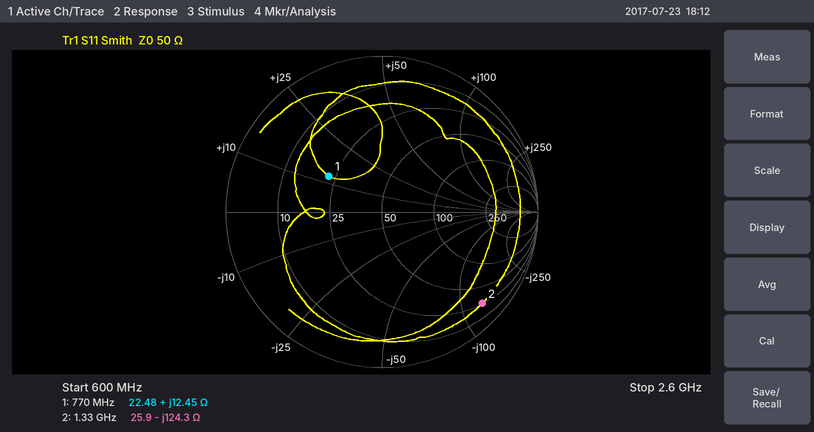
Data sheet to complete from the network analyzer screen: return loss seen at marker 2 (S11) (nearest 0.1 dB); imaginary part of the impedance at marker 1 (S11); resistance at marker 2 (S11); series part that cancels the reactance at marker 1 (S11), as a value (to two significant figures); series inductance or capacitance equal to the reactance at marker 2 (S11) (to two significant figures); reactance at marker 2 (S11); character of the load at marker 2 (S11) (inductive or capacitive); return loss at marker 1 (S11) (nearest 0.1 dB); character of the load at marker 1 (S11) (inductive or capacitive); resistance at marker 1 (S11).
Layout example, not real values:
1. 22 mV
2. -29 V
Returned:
1. 1.2 dB
2. +12.45 Ω
3. 25.9 Ω
4. 17 pF
5. 960 fF
6. -124.3 Ω
7. capacitive
8. 7.7 dB
9. inductive
10. 22.48 Ω
